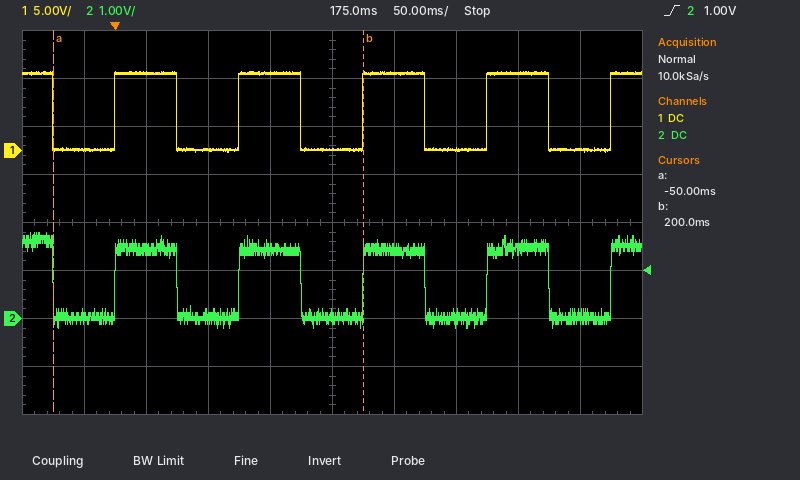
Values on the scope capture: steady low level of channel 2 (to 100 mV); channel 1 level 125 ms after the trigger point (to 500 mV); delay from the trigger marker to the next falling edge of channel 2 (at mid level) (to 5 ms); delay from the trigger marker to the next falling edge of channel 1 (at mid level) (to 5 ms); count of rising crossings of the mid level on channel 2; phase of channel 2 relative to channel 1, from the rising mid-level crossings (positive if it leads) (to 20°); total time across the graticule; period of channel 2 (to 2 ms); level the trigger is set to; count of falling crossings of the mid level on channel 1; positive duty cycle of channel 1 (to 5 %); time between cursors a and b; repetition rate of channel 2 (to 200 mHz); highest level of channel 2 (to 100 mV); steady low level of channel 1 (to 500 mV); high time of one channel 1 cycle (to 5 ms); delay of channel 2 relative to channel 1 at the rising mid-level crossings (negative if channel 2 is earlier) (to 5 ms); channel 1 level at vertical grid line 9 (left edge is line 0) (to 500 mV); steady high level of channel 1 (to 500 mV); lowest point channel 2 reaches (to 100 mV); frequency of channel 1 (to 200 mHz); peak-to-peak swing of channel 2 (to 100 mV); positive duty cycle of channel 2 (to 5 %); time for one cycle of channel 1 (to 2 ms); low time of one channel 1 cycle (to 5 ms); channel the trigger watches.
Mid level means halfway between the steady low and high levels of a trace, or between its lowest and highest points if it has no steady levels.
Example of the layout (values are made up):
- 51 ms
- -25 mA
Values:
- 0.0 V
- 8.0 V
- 50 ms
- 50 ms
- 5
- 0°
- 500 ms
- 100 ms
- 1.00 V
- 5
- 50 %
- 250 ms
- 10.0 Hz
- 1.8 V
- 0.0 V
- 50 ms
- 0 ms
- 0.0 V
- 8.0 V
- -200 mV
- 10.0 Hz
- 2.0 V
- 50 %
- 100 ms
- 50 ms
- channel 2
